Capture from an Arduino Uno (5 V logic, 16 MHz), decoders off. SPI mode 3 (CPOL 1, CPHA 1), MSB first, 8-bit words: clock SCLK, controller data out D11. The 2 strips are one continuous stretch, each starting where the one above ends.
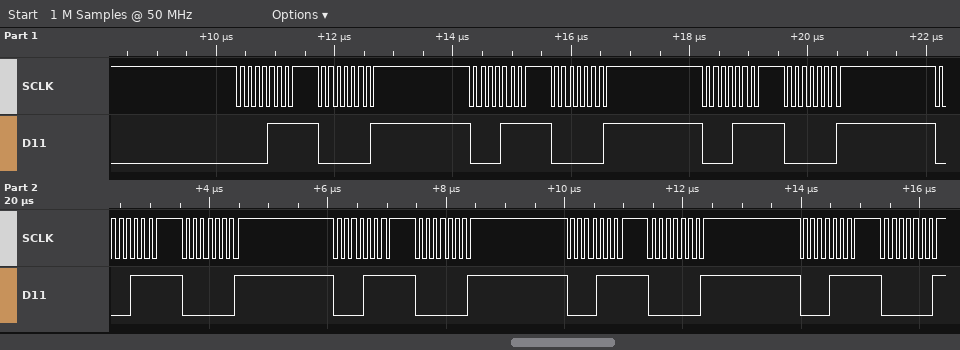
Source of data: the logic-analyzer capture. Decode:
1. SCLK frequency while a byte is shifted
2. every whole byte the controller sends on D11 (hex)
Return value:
8 MHz
0F 01 0F 01 0F 01 0F 01 0F 01 0F 01 0F 01
